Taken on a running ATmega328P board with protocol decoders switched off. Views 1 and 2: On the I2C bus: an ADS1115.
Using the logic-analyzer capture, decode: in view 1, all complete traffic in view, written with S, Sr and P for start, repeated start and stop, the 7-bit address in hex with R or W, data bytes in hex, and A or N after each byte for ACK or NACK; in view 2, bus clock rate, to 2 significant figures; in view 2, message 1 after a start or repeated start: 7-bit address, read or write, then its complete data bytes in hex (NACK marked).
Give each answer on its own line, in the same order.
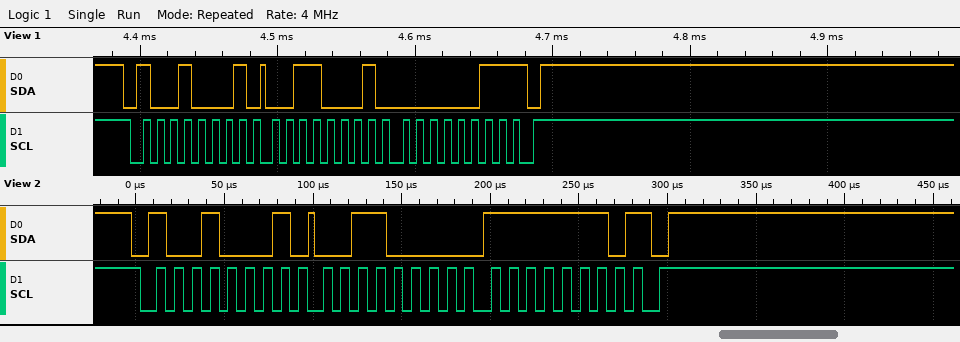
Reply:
S 48R A 31 A 03 N P
100 kHz
0x48 read: 30 FE NACK
